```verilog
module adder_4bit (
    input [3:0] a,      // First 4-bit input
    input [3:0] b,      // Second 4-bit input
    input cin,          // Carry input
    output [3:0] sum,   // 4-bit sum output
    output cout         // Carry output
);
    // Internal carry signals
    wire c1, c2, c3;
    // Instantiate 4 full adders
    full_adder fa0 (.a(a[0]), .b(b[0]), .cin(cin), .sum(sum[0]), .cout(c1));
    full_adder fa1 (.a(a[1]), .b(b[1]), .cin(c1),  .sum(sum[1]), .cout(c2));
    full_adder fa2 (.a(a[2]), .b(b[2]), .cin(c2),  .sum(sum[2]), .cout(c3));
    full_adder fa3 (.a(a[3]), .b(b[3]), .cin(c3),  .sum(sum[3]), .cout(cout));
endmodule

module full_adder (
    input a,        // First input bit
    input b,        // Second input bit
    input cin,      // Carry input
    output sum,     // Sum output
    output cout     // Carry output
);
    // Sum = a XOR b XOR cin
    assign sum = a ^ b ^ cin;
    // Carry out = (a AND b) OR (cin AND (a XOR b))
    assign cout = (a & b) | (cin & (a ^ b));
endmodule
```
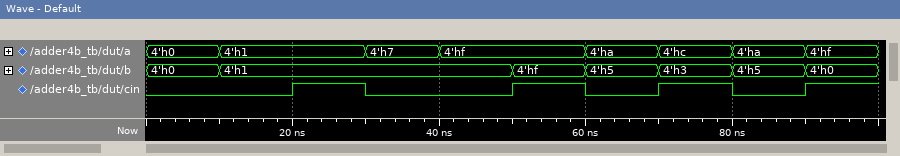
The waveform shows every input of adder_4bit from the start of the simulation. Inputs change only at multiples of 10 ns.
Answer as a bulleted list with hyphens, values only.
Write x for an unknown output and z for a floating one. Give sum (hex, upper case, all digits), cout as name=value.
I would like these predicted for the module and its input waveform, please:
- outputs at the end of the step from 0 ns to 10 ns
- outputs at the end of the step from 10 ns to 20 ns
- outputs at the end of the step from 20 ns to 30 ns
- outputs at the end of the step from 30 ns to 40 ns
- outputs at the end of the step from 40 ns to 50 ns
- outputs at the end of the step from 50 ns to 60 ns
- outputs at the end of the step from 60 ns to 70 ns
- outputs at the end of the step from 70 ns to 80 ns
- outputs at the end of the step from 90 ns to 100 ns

- sum=0, cout=0
- sum=2, cout=0
- sum=3, cout=0
- sum=8, cout=0
- sum=0, cout=1
- sum=F, cout=1
- sum=F, cout=0
- sum=0, cout=1
- sum=0, cout=1
